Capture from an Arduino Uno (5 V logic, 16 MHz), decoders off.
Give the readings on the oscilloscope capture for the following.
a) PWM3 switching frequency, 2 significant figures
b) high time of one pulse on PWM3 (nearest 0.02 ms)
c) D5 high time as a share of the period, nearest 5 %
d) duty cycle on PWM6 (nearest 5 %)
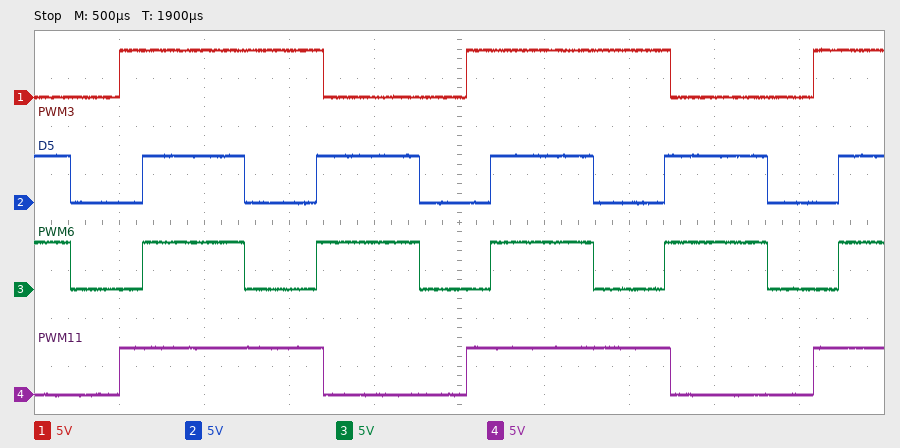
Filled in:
490 Hz
1.20 ms
60 %
60 %
